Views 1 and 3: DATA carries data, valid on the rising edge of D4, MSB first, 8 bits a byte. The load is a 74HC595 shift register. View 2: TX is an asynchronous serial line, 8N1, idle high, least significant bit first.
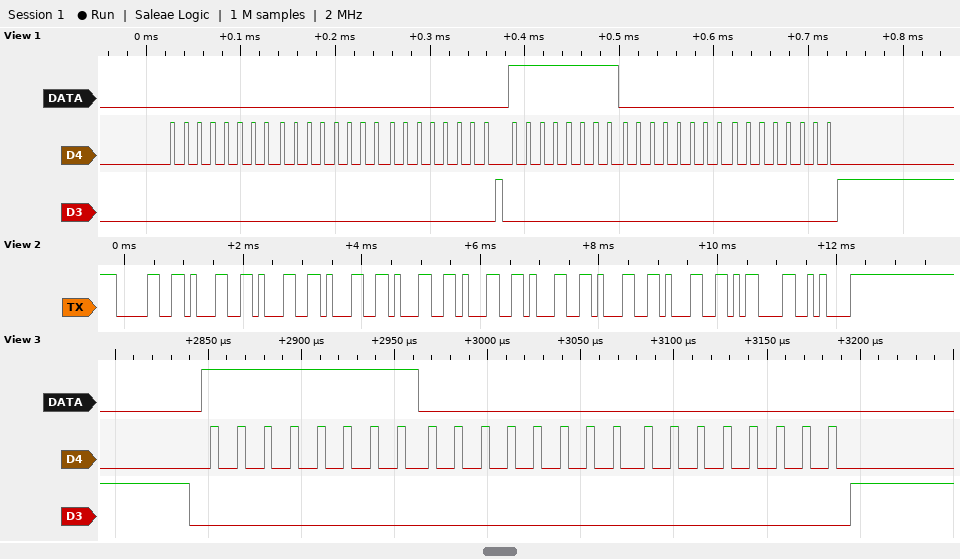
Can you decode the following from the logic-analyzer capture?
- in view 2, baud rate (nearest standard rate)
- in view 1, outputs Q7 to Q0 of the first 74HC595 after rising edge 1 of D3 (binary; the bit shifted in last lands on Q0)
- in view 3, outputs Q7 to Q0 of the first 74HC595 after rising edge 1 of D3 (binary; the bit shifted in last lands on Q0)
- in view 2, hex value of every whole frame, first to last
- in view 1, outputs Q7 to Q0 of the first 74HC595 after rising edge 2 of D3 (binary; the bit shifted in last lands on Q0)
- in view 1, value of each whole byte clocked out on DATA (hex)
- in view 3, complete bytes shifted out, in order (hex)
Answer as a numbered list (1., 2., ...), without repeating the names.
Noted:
1. 9600 baud
2. 00000000
3. 00000000
4. 30 31 31 31 31 31 31 31 31 0D 0A
5. 00000000
6. 00 00 00 FF 00 00
7. FF 00 00
